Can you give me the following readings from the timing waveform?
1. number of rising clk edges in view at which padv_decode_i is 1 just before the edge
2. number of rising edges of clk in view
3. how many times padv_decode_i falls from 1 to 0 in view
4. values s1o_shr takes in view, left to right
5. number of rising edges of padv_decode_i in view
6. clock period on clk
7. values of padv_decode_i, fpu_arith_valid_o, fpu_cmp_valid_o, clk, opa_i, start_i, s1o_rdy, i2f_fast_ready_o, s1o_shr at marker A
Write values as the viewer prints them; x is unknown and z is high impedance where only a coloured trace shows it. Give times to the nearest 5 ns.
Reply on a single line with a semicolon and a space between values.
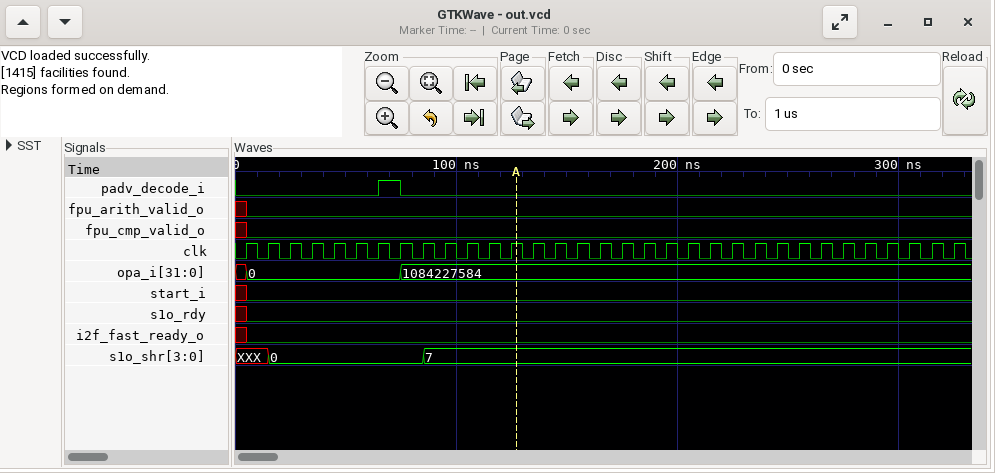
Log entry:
1; 33; 1; XXX, 0, 7; 1; 10 ns; padv_decode_i=0, fpu_arith_valid_o=0, fpu_cmp_valid_o=0, clk=1, opa_i=1084227584, start_i=0, s1o_rdy=0, i2f_fast_ready_o=0, s1o_shr=7
